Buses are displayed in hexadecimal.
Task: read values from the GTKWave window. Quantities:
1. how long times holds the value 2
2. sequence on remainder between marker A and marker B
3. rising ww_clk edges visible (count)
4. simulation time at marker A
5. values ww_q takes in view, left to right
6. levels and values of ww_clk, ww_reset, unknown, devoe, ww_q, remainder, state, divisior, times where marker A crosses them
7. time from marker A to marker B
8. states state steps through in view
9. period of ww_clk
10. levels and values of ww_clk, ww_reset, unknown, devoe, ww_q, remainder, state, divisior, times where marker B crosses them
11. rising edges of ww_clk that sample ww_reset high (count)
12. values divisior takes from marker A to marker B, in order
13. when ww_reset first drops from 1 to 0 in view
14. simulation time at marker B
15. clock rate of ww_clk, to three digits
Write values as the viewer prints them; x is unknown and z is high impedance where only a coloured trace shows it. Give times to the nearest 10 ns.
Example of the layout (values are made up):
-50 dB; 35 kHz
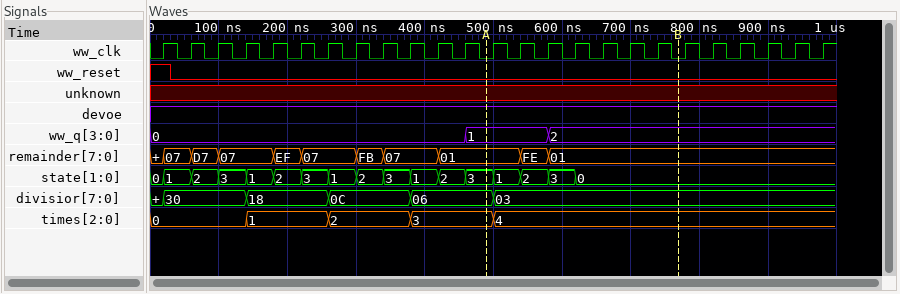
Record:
120 ns; 01, FE, 01; 25; 490 ns; 0, 1, 2; ww_clk=0, ww_reset=0, unknown=x, devoe=1, ww_q=1, remainder=01, state=3, divisior=06, times=3; 280 ns; 0, 1, 2, 3, 1, 2, 3, 1, 2, 3, 1, 2, 3, 1, 2, 3, 0; 40 ns; ww_clk=0, ww_reset=0, unknown=x, devoe=1, ww_q=2, remainder=01, state=0, divisior=03, times=4; 1; 06, 03; 30 ns; 770 ns; 25.0 MHz
